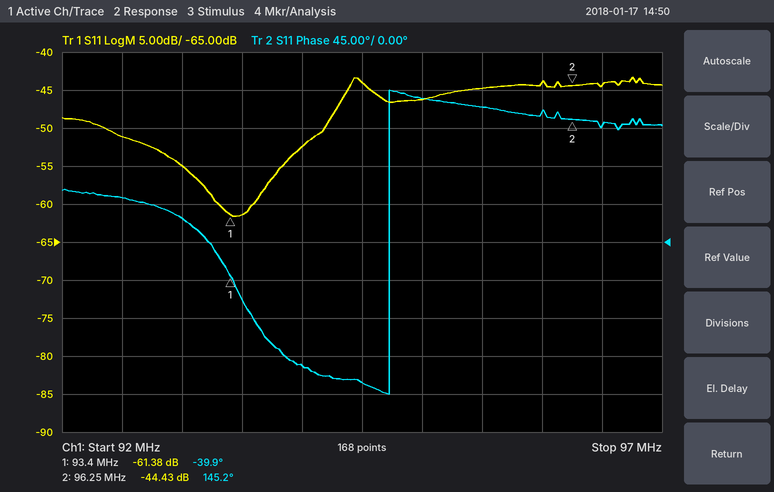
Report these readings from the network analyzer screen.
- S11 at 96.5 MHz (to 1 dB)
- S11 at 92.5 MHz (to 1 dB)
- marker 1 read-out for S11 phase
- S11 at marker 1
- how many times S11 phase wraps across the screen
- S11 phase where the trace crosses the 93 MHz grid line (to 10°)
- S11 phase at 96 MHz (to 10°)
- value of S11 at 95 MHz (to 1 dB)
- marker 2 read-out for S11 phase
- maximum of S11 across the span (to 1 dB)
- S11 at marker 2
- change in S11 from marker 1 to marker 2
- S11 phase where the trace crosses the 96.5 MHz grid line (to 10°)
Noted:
-44 dB
-51 dB
-39.9°
-61.38 dB
1
30°
150°
-46 dB
145.2°
-43 dB
-44.43 dB
16.95 dB
140°
